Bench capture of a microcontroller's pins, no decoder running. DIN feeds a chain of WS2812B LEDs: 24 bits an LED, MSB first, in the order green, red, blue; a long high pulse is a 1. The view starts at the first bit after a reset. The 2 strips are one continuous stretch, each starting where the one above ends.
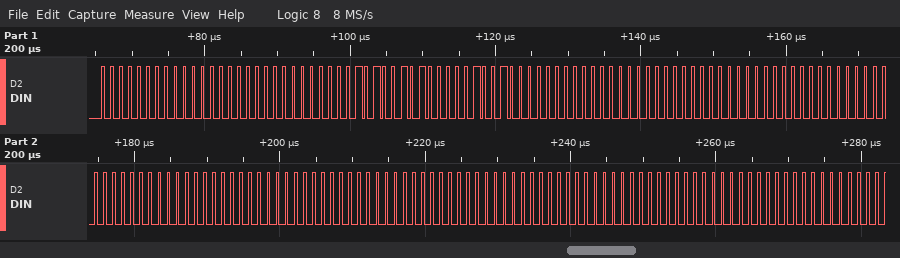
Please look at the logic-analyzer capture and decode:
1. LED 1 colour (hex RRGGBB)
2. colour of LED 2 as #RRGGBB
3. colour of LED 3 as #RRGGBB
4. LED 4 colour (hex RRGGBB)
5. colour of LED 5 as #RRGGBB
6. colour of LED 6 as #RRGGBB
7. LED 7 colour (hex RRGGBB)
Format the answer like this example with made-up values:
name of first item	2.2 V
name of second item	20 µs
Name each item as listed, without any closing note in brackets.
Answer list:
LED 1 colour	#000000
colour of LED 2 as #RRGGBB	#500A48
colour of LED 3 as #RRGGBB	#000000
LED 4 colour	#000000
colour of LED 5 as #RRGGBB	#000000
colour of LED 6 as #RRGGBB	#000000
LED 7 colour	#000000
